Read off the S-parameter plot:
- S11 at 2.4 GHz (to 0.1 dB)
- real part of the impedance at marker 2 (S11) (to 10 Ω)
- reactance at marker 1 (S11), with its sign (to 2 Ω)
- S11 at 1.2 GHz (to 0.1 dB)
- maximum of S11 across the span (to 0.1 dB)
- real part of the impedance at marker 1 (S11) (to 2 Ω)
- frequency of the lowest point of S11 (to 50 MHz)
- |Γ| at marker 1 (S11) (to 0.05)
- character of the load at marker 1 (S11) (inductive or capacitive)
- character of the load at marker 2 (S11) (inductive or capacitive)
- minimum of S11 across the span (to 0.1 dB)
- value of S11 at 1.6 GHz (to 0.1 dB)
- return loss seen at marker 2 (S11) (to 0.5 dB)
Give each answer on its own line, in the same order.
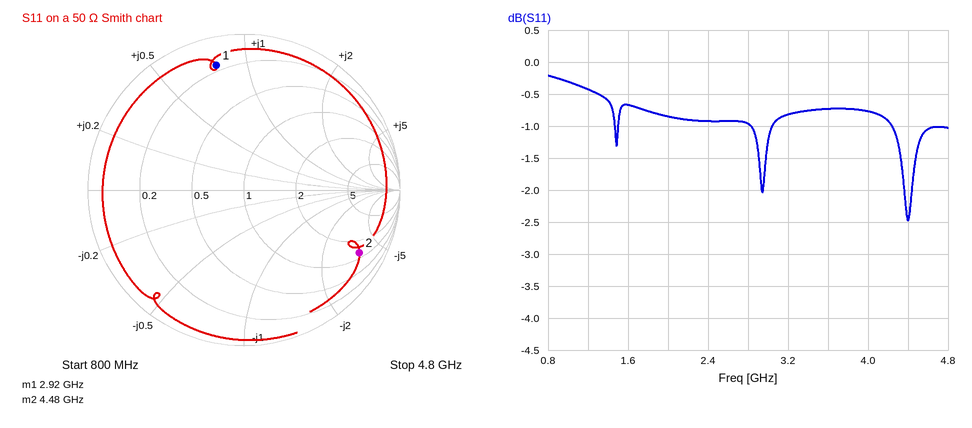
-0.9 dB
60 Ω
+40 Ω
-0.4 dB
-0.2 dB
8 Ω
4.40 GHz
0.80
inductive
capacitive
-2.5 dB
-0.7 dB
1.5 dB
